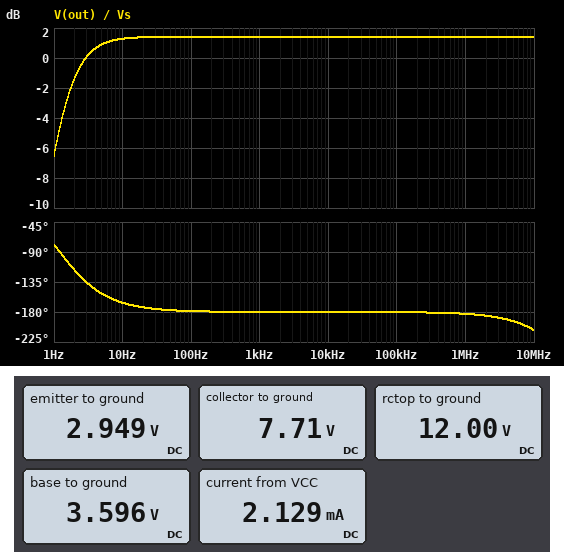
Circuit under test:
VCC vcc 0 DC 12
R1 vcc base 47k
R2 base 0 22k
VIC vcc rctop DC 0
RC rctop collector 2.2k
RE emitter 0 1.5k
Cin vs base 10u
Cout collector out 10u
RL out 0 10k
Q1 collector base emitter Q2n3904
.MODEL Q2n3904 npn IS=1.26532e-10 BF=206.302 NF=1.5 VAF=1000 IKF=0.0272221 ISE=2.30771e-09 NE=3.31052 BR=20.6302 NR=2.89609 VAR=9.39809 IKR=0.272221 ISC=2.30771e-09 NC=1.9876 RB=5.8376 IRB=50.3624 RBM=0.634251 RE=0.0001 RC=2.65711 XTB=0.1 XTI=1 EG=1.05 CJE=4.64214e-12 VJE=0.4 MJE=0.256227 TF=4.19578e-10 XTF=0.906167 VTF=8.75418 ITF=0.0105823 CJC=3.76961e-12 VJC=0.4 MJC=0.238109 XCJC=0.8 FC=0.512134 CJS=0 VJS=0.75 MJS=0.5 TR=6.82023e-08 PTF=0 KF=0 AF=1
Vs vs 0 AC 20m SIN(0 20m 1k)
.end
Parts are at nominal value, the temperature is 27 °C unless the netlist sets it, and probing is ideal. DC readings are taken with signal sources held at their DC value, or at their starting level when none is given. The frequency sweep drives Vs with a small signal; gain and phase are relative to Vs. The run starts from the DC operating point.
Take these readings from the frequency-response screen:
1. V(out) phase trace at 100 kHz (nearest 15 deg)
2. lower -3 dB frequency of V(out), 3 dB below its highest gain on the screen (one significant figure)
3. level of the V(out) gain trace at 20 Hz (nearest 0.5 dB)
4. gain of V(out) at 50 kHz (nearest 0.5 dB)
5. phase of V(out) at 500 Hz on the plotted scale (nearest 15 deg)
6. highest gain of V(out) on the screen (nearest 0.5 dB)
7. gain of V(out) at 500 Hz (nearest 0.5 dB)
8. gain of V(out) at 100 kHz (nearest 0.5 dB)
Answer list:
-180 deg
2 Hz
1.5 dB
1.5 dB
-180 deg
1.5 dB
1.5 dB
1.5 dB
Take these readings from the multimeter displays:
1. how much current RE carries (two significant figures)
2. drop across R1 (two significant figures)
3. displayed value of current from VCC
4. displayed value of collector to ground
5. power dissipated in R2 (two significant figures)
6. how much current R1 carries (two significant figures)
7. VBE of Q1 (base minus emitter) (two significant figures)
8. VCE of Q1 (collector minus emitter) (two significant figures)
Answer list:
2.0 mA
8.4 V
2.129 mA
7.71 V
590 µW
180 µA
650 mV
4.8 V
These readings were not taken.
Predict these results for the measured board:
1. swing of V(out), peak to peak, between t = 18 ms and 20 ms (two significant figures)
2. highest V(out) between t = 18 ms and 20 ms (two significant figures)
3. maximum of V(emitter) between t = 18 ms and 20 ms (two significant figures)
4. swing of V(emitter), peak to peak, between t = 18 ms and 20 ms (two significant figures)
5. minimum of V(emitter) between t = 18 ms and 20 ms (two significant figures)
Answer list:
47 mV
24 mV
3.0 V
39 mV
2.9 V
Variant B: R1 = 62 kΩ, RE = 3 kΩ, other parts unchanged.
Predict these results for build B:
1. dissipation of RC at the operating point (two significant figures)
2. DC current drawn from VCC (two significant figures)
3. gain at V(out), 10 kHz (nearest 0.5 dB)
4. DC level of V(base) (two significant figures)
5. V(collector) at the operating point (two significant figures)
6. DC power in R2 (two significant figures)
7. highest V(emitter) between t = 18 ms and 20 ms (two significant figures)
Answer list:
1.4 mW
940 µA
-4.5 dB
3.0 V
10 V
420 µW
2.4 V
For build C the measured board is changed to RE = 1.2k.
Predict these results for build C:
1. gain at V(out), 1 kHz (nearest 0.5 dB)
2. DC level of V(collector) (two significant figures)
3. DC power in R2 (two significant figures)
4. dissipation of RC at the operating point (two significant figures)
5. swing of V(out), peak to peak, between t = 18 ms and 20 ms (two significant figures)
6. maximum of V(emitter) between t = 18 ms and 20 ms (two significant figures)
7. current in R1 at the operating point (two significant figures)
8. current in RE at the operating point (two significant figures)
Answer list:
3.5 dB
6.7 V
570 µW
13 mW
59 mV
2.9 V
180 µA
2.4 mA
